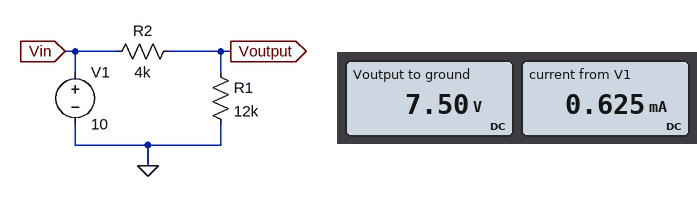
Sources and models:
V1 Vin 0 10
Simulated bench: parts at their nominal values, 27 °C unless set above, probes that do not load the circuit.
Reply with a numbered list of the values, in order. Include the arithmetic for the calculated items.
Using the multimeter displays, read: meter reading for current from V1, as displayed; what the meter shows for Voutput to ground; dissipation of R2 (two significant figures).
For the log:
1. 0.625 mA
2. 7.50 V
3. (10 V - 7.5 V)^2 / 4 kΩ = 1.6 mW
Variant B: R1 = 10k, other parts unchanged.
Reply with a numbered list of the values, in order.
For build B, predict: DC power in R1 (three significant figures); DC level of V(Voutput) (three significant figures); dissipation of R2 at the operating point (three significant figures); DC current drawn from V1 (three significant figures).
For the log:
1. 5.10 mW
2. 7.14 V
3. 2.04 mW
4. 714 µA
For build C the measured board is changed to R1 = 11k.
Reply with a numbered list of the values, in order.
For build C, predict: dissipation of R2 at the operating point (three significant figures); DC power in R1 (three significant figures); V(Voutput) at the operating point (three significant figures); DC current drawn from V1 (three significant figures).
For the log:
1. 1.78 mW
2. 4.89 mW
3. 7.33 V
4. 667 µA
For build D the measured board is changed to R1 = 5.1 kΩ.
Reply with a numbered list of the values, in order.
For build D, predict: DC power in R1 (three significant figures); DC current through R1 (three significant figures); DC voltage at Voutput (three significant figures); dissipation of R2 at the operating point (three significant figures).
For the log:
1. 6.16 mW
2. 1.10 mA
3. 5.60 V
4. 4.83 mW
